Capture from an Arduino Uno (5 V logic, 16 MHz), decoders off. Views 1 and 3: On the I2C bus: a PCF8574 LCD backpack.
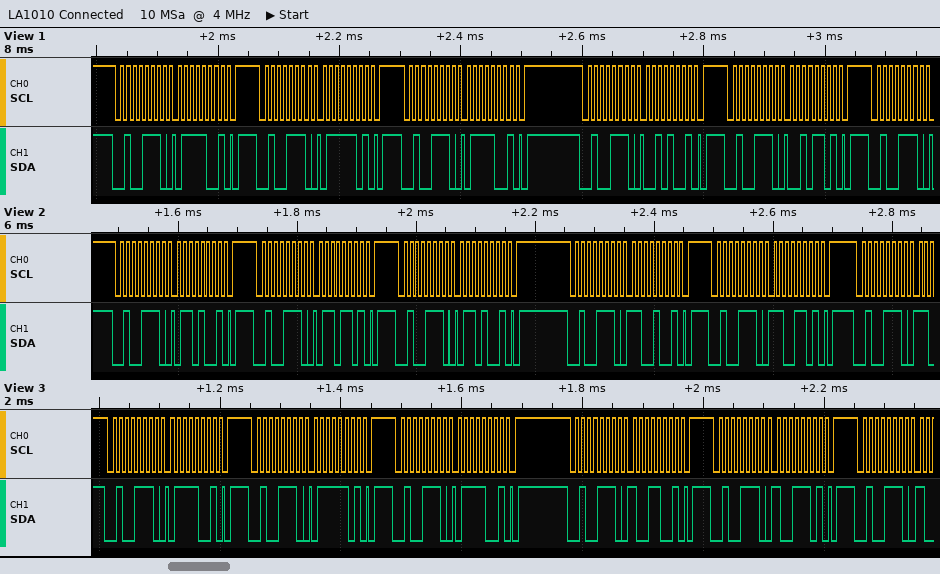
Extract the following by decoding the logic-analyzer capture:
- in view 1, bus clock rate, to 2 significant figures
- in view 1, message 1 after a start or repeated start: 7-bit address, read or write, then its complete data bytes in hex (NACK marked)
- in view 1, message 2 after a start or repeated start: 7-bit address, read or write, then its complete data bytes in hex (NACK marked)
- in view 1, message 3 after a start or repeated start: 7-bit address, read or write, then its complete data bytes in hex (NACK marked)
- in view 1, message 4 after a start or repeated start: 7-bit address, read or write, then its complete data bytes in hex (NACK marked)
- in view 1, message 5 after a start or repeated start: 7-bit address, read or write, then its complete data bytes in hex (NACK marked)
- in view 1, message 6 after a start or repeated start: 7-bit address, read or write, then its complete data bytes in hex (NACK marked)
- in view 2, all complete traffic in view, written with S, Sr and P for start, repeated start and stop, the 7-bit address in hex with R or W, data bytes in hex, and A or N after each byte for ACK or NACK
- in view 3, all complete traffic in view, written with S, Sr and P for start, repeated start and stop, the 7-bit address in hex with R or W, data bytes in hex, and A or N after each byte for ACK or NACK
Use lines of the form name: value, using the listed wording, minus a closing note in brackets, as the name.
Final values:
in view 1, bus clock rate, to 2 significant figures: 100 kHz
in view 1, message 1 after a start or repeated start: 7-bit address, read or write, then its complete data bytes in hex: 0x27 write: 79
in view 1, message 2 after a start or repeated start: 7-bit address, read or write, then its complete data bytes in hex: 0x27 write: 7D
in view 1, message 3 after a start or repeated start: 7-bit address, read or write, then its complete data bytes in hex: 0x27 write: 79
in view 1, message 4 after a start or repeated start: 7-bit address, read or write, then its complete data bytes in hex: 0x27 write: 29
in view 1, message 5 after a start or repeated start: 7-bit address, read or write, then its complete data bytes in hex: 0x27 write: 2D
in view 1, message 6 after a start or repeated start: 7-bit address, read or write, then its complete data bytes in hex: 0x27 write
in view 2, all complete traffic in view, written with S, Sr and P for start, repeated start and stop, the 7-bit address in hex with R or W, data bytes in hex, and A or N after each byte for ACK or NACK: S 27W A 69 A P S 27W A 6D A P S 27W A 69 A P S 27W A C9 A P S 27W A CD A P S 27W A
in view 3, all complete traffic in view, written with S, Sr and P for start, repeated start and stop, the 7-bit address in hex with R or W, data bytes in hex, and A or N after each byte for ACK or NACK: S 27W A 79 A P S 27W A 7D A P S 27W A 79 A P S 27W A 99 A P S 27W A 9D A P S 27W A
